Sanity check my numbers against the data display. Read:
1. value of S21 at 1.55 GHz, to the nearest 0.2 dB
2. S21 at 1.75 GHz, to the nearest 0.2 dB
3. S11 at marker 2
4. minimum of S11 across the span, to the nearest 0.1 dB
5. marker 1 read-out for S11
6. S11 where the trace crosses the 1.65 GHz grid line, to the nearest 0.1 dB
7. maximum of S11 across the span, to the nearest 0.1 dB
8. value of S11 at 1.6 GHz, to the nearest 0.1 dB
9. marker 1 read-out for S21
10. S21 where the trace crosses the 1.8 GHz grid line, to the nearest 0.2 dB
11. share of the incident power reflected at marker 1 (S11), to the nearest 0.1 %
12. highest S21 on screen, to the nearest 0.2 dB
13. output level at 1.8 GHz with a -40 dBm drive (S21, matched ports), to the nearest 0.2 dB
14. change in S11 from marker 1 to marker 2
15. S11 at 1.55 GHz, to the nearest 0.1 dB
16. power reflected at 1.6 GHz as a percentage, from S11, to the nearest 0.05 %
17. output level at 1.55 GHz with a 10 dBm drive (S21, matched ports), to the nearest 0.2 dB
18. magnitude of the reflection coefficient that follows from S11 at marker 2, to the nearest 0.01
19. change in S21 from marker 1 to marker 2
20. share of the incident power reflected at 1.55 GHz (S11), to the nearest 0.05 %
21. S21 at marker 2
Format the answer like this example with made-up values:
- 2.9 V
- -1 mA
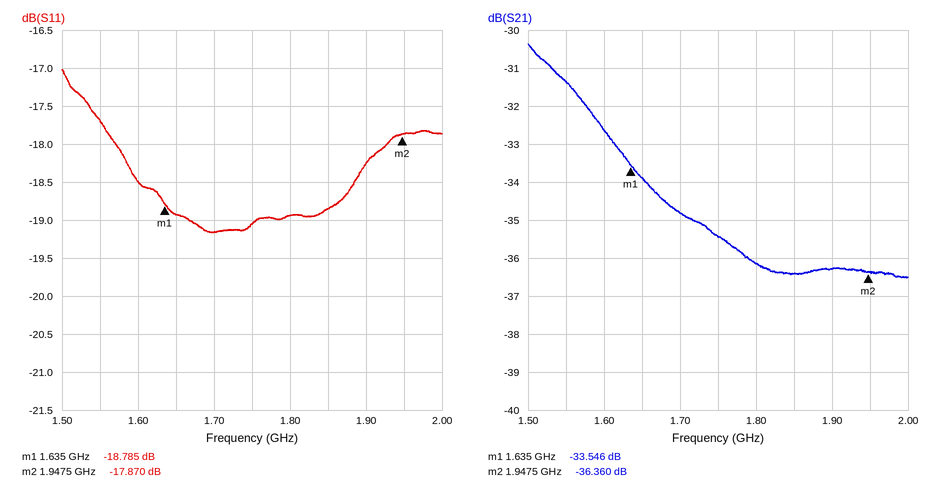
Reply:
- -31.4 dB
- -35.4 dB
- -17.870 dB
- -19.2 dB
- -18.785 dB
- -18.9 dB
- -17.0 dB
- -18.5 dB
- -33.546 dB
- -36.2 dB
- 1.3 %
- -30.4 dB
- -76.2 dBm
- 0.915 dB
- -17.7 dB
- 1.40 %
- -21.4 dBm
- 0.13
- -2.814 dB
- 1.70 %
- -36.360 dB
